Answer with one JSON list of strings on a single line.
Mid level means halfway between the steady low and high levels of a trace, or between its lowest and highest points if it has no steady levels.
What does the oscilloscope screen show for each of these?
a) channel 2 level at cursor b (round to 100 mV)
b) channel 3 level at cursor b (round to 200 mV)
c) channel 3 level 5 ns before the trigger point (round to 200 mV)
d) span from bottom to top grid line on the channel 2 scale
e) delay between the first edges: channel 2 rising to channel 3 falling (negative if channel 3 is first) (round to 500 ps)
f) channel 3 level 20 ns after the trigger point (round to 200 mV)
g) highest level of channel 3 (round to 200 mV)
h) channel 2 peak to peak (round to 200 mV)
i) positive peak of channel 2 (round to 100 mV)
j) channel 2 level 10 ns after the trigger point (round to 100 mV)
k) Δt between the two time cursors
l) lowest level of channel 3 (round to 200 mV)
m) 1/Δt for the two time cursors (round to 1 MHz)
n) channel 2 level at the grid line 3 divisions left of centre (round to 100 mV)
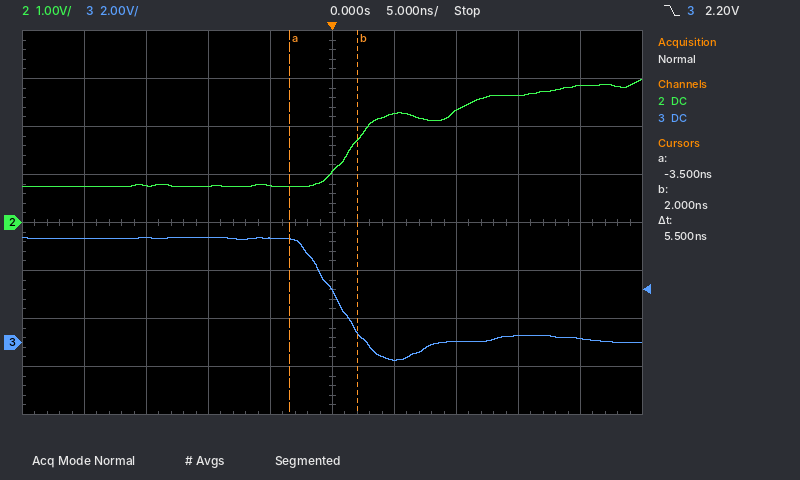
["1.7 V", "400 mV", "4.4 V", "8 V", "-2.0 ns", "200 mV", "4.4 V", "2.2 V", "3.0 V", "2.3 V", "5.5 ns", "-800 mV", "182 MHz", "800 mV"]
